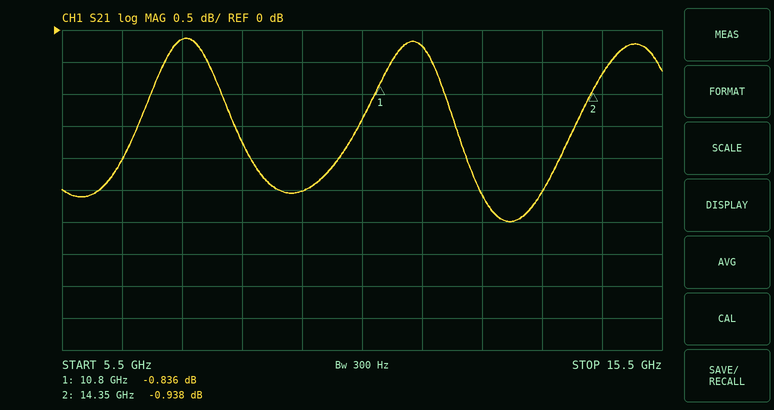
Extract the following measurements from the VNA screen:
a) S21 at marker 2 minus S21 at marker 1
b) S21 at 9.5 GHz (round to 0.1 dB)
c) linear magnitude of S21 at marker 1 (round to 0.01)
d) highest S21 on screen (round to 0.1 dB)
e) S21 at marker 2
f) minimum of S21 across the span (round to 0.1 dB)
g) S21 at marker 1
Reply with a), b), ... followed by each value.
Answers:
a) -0.102 dB
b) -2.5 dB
c) 0.91
d) -0.1 dB
e) -0.938 dB
f) -3.0 dB
g) -0.836 dB
